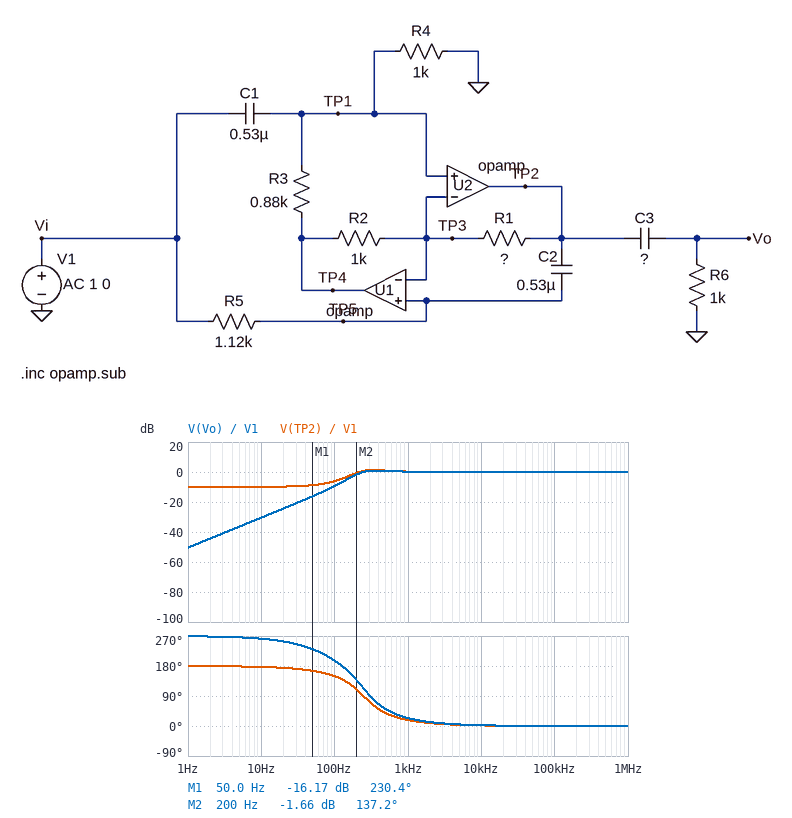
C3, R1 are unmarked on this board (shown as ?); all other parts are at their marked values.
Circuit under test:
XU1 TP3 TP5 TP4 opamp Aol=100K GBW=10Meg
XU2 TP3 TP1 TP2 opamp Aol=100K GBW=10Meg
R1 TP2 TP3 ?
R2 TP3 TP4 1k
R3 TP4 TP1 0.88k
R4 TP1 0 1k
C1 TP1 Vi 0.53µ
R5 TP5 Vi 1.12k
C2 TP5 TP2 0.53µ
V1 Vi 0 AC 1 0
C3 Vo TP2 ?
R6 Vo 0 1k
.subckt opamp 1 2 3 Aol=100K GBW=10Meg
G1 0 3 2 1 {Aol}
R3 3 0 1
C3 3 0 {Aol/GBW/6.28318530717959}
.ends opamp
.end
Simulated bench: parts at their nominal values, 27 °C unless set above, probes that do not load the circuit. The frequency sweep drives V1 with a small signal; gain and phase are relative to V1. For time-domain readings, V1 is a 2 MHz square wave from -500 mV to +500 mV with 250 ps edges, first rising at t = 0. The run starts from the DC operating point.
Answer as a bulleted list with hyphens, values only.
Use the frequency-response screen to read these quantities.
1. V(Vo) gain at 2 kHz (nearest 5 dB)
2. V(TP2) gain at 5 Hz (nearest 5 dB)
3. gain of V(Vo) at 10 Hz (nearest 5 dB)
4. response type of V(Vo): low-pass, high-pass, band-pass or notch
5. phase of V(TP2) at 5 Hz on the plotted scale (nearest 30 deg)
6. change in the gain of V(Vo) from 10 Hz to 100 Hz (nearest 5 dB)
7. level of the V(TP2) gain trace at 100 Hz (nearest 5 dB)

- 0 dB
- -10 dB
- -30 dB
- high-pass
- 180 deg
- 20 dB
- -5 dB
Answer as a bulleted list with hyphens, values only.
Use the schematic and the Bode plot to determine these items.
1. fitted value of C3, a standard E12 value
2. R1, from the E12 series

- 1.5 µF
- 1.5 kΩ
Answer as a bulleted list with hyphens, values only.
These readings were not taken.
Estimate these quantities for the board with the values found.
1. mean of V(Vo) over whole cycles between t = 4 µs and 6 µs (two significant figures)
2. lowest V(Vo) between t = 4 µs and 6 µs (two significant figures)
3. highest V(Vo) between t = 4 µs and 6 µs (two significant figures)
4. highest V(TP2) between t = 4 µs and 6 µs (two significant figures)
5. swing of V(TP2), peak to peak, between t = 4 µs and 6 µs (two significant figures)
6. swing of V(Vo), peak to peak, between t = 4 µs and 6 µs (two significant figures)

- 490 mV
- -240 mV
- 1.2 V
- 1.4 V
- 1.5 V
- 1.5 V
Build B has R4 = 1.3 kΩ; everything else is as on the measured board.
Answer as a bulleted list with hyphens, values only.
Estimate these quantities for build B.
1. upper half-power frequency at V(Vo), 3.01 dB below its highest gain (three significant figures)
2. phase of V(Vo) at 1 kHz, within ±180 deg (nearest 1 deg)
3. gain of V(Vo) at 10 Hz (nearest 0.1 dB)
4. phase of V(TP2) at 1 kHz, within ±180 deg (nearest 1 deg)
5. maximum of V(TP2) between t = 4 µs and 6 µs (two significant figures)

- 11.8 MHz
- 20 deg
- -55.9 dB
- 14 deg
- 1.2 V
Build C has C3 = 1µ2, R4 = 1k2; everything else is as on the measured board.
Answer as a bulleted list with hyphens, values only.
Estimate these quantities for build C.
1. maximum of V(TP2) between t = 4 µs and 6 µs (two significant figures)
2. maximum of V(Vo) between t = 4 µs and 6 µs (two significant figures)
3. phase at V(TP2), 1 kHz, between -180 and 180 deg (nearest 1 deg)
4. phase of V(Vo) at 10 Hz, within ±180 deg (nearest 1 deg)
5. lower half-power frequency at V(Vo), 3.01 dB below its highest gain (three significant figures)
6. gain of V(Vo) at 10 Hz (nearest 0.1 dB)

- 1.3 V
- 1.2 V
- 15 deg
- -97 deg
- 241 Hz
- -42.3 dB
